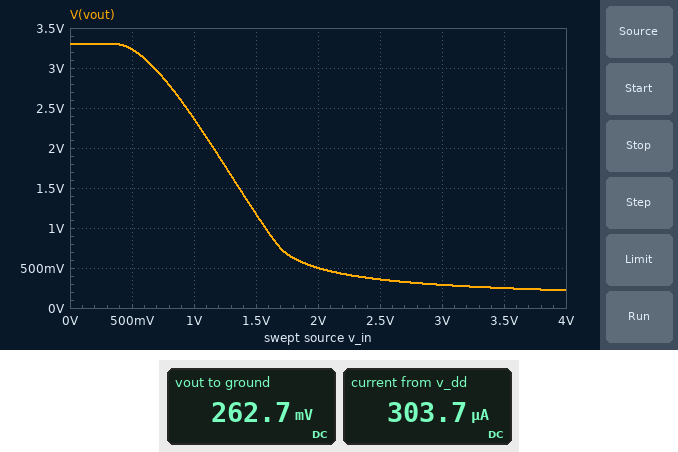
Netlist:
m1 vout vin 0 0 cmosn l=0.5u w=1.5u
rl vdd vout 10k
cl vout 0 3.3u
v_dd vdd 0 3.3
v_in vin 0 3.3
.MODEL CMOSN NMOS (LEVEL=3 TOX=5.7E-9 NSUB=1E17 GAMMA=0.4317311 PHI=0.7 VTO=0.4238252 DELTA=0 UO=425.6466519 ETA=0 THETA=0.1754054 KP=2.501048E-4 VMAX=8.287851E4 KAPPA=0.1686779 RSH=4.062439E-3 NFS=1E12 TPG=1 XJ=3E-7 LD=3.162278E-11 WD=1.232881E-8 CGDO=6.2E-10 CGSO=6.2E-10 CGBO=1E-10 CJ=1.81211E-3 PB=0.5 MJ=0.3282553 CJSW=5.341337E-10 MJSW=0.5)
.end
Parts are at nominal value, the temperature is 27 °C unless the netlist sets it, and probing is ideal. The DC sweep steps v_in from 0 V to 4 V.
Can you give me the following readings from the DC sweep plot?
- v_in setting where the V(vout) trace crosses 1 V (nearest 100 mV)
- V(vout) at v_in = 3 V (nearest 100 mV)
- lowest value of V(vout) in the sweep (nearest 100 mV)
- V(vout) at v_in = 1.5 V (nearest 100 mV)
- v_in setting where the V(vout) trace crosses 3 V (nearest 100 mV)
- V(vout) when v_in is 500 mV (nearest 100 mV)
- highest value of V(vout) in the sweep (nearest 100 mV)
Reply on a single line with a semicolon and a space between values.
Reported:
1.6 V; 300 mV; 200 mV; 1.2 V; 700 mV; 3.2 V; 3.3 V
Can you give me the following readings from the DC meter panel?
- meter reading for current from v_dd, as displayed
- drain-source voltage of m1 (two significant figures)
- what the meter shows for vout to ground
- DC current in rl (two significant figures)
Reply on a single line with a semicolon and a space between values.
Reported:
303.7 µA; 260 mV; 262.7 mV; 300 µA
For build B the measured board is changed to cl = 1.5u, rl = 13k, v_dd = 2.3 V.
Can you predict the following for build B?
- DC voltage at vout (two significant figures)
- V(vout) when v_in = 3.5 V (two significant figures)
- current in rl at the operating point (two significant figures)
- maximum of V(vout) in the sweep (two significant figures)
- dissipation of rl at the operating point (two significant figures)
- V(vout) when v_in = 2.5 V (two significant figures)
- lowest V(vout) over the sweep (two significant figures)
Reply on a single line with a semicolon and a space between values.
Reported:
130 mV; 120 mV; 170 µA; 2.3 V; 360 µW; 170 mV; 110 mV
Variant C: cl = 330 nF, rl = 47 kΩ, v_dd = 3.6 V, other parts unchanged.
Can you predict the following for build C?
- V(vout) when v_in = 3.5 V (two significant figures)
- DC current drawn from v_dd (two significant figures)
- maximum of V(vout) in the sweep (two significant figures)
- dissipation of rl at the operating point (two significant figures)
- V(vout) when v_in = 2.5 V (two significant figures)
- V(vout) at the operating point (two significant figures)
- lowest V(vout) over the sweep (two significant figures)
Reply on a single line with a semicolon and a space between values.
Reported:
53 mV; 75 µA; 3.6 V; 270 µW; 70 mV; 55 mV; 48 mV
